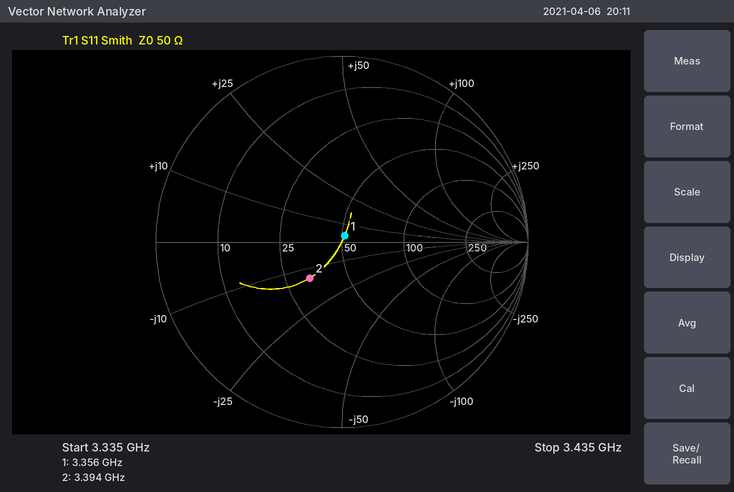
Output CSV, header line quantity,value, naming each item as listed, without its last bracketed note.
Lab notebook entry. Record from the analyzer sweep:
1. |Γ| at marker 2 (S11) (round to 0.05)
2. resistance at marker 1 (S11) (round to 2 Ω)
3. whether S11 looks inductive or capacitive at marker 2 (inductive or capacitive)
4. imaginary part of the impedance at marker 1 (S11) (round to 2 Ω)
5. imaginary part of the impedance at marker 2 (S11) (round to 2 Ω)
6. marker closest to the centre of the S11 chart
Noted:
quantity,value
|Γ| at marker 2 (S11),0.25
resistance at marker 1 (S11),52 Ω
whether S11 looks inductive or capacitive at marker 2,capacitive
imaginary part of the impedance at marker 1 (S11),+4 Ω
imaginary part of the impedance at marker 2 (S11),-14 Ω
marker closest to the centre of the S11 chart,marker 1
